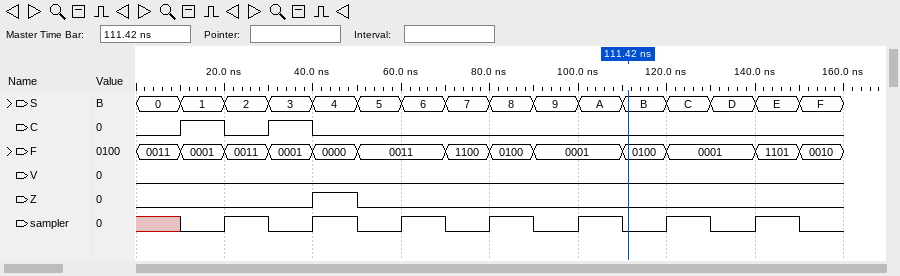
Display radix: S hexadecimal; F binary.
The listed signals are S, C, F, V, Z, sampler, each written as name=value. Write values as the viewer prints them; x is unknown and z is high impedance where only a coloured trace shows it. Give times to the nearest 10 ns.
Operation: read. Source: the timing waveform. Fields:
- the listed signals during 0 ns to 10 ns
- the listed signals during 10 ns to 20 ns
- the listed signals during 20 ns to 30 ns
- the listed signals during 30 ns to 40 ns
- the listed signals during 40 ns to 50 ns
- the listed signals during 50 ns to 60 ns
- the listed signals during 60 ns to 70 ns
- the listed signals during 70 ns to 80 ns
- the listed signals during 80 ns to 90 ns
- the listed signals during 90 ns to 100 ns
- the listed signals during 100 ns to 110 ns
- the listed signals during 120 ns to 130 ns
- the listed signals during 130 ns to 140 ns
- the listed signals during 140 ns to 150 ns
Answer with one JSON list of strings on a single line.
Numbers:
["S=0, C=0, F=0011, V=0, Z=0, sampler=x", "S=1, C=1, F=0001, V=0, Z=0, sampler=0", "S=2, C=0, F=0011, V=0, Z=0, sampler=1", "S=3, C=1, F=0001, V=0, Z=0, sampler=0", "S=4, C=0, F=0000, V=0, Z=1, sampler=1", "S=5, C=0, F=0011, V=0, Z=0, sampler=0", "S=6, C=0, F=0011, V=0, Z=0, sampler=1", "S=7, C=0, F=1100, V=0, Z=0, sampler=0", "S=8, C=0, F=0100, V=0, Z=0, sampler=1", "S=9, C=0, F=0001, V=0, Z=0, sampler=0", "S=A, C=0, F=0001, V=0, Z=0, sampler=1", "S=C, C=0, F=0001, V=0, Z=0, sampler=1", "S=D, C=0, F=0001, V=0, Z=0, sampler=0", "S=E, C=0, F=1101, V=0, Z=0, sampler=1"]
